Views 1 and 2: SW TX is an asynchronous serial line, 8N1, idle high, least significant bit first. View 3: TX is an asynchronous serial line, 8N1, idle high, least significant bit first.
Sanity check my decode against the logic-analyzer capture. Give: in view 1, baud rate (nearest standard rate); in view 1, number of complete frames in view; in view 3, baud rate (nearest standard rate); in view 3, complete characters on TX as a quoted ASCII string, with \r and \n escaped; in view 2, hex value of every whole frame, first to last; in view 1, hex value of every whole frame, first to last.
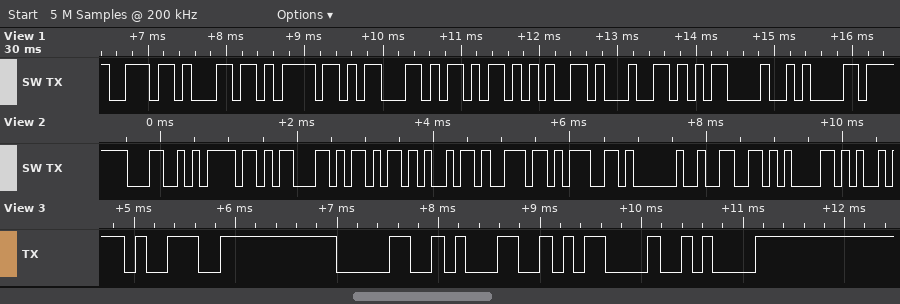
9600 baud
9
9600 baud
"901\r\n"
0x4C 0x6F 0x63 0x6B 0x69 0x6E 0x67 0x20 0x66 0x61
0x6E 0x6C 0x6F 0x63 0x6B 0x65 0x64 0x0D 0x0A
